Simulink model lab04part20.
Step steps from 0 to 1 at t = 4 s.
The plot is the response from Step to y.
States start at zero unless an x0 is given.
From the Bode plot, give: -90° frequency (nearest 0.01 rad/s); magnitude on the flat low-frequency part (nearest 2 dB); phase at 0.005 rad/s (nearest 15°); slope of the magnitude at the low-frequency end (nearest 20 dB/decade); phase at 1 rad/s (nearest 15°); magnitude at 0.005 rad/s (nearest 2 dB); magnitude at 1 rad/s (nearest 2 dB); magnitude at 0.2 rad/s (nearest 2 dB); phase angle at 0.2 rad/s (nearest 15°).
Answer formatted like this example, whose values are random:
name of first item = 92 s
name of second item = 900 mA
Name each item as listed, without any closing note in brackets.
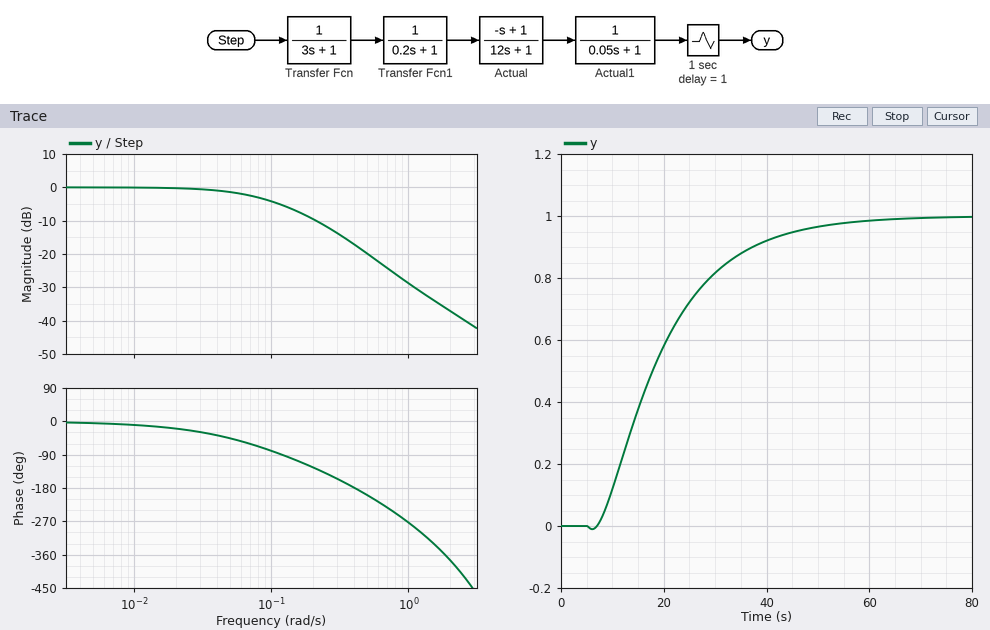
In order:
-90° frequency = 0.12 rad/s
magnitude on the flat low-frequency part = 0 dB
phase at 0.005 rad/s = 0°
slope of the magnitude at the low-frequency end = 0 dB/decade
phase at 1 rad/s = -270°
magnitude at 0.005 rad/s = 0 dB
magnitude at 1 rad/s = -28 dB
magnitude at 0.2 rad/s = -10 dB
phase angle at 0.2 rad/s = -120°
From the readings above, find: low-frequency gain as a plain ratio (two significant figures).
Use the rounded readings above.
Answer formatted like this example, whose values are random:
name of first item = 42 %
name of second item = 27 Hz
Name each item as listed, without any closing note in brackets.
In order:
low-frequency gain as a plain ratio = 1.0
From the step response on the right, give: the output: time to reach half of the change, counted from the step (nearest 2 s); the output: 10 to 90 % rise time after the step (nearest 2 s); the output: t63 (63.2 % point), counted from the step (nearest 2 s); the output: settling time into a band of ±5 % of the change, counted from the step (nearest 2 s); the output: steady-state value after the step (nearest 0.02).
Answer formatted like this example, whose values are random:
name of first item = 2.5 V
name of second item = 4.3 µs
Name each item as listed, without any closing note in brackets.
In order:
the output: time to reach half of the change, counted from the step = 14 s
the output: 10 to 90 % rise time after the step = 28 s
the output: t63 (63.2 % point), counted from the step = 18 s
the output: settling time into a band of ±5 % of the change, counted from the step = 42 s
the output: steady-state value after the step = 1.00
